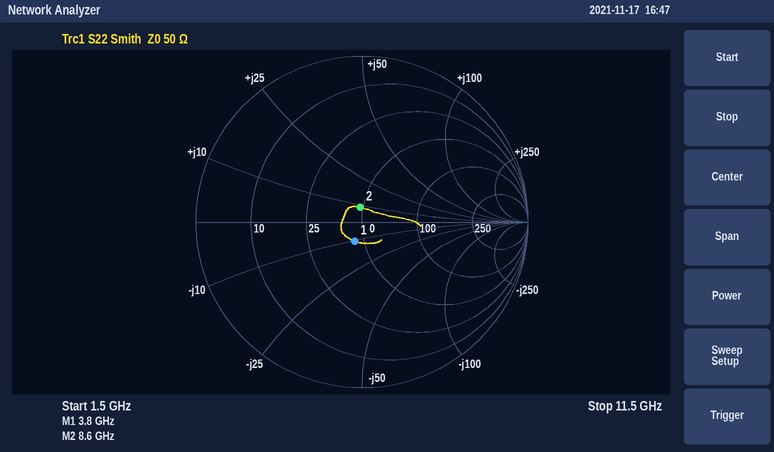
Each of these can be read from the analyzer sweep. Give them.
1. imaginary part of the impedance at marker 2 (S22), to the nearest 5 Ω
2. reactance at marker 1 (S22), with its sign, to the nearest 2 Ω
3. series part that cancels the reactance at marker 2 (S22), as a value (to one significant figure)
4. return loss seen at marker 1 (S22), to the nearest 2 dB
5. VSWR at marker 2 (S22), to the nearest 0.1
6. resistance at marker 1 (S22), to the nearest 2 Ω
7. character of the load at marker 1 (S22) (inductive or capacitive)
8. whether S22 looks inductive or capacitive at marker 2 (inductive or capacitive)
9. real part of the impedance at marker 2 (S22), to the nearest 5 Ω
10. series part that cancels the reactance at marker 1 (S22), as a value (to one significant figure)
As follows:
+10 Ω
-10 Ω
2 pF
18 dB
1.2
44 Ω
capacitive
inductive
50 Ω
400 pH
